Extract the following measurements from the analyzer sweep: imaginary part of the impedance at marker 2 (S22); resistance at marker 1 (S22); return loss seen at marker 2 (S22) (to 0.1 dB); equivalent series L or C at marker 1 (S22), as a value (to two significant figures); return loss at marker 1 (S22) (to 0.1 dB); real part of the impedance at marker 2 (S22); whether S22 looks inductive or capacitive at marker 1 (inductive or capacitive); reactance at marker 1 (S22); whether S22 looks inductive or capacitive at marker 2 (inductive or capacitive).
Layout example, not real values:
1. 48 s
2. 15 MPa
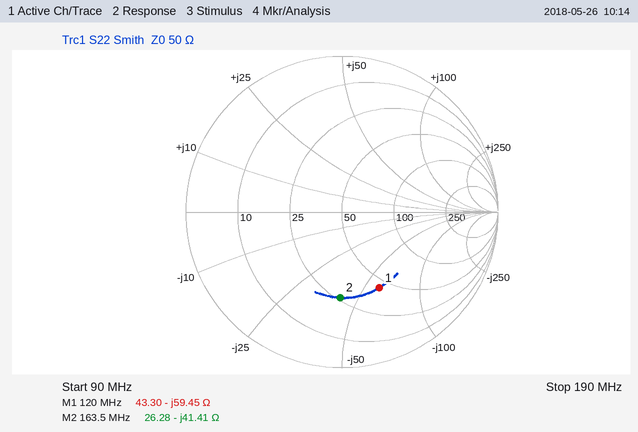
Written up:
1. -41.41 Ω
2. 43.30 Ω
3. 5.2 dB
4. 22 pF
5. 5.3 dB
6. 26.28 Ω
7. capacitive
8. -59.45 Ω
9. capacitive
